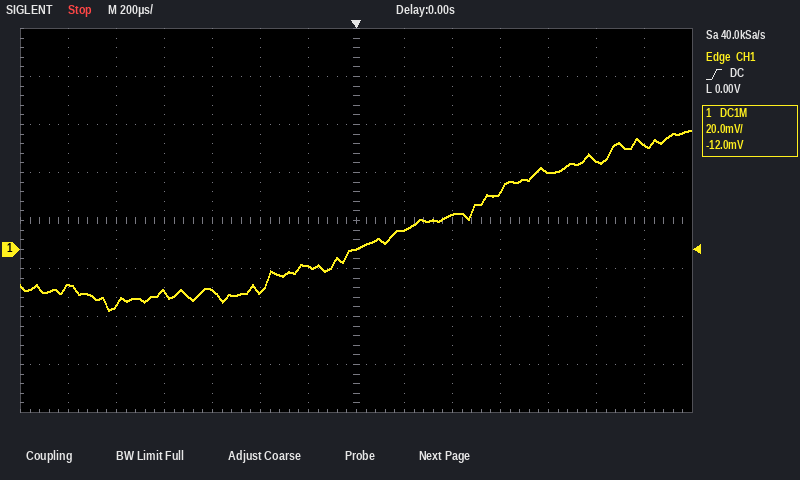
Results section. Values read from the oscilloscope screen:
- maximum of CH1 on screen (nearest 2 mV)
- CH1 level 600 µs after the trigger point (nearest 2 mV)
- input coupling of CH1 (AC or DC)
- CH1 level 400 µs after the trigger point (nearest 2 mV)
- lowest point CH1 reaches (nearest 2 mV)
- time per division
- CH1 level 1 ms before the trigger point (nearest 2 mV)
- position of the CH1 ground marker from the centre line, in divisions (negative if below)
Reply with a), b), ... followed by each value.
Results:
a) 50 mV
b) 24 mV
c) DC
d) 14 mV
e) -26 mV
f) 200 µs
g) -24 mV
h) -0.6 div
